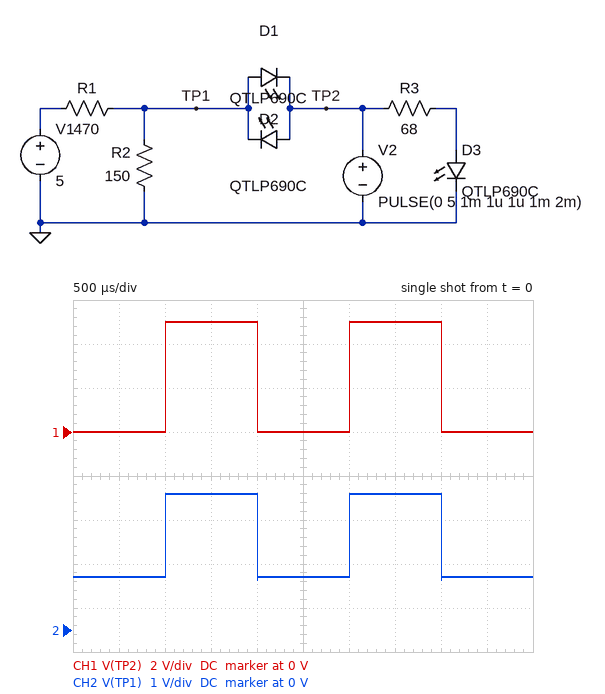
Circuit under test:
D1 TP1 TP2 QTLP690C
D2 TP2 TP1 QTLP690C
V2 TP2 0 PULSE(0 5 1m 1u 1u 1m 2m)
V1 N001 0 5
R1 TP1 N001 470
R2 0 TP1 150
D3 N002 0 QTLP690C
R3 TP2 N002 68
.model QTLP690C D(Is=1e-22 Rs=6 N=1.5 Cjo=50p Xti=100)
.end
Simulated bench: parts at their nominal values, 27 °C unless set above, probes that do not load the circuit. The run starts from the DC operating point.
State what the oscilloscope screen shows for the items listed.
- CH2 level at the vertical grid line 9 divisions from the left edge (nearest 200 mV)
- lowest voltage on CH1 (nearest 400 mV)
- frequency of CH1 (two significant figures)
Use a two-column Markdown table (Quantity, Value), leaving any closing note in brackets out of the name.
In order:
| Quantity | Value |
|---|---|
| CH2 level at the vertical grid line 9 divisions from the left edge | 1.2 V |
| lowest voltage on CH1 | 0 V |
| frequency of CH1 | 500 Hz |
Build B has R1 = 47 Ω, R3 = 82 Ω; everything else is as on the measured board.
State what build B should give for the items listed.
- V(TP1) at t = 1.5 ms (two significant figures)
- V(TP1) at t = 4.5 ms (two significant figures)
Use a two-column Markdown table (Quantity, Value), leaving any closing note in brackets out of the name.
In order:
| Quantity | Value |
|---|---|
| V(TP1) at t = 1.5 ms | 3.8 V |
| V(TP1) at t = 4.5 ms | 2.1 V |
